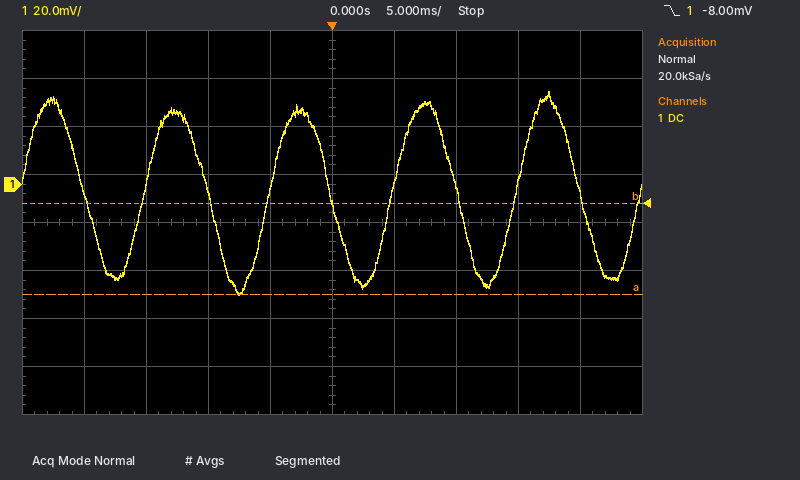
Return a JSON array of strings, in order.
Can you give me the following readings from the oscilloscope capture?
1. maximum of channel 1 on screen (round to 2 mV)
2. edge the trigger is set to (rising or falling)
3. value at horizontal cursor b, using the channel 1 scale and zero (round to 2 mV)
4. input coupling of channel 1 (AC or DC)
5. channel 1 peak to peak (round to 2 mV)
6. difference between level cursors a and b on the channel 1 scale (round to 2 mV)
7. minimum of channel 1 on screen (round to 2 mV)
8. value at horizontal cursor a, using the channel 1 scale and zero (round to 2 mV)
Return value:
["38 mV", "falling", "-8 mV", "DC", "84 mV", "38 mV", "-46 mV", "-46 mV"]
